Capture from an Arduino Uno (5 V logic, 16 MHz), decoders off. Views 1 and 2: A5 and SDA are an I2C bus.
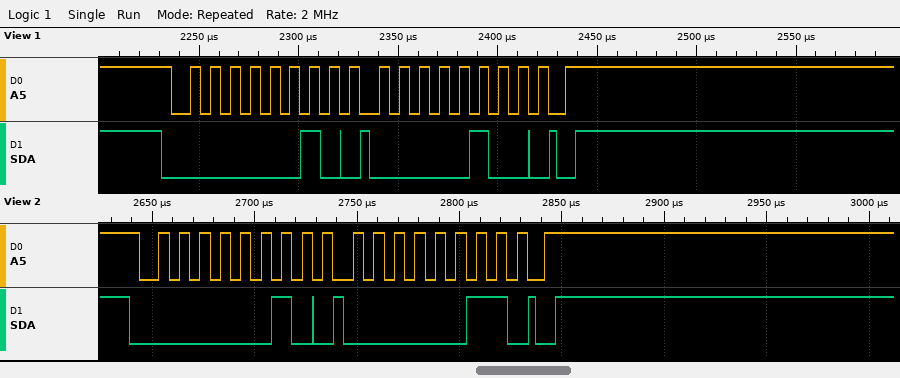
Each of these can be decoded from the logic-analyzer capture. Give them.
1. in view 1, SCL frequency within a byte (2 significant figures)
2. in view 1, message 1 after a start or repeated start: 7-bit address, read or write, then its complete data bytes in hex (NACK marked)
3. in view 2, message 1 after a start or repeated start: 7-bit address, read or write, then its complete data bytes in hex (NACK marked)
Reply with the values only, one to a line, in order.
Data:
100 kHz
0x01 write: 04
0x01 write: 03
